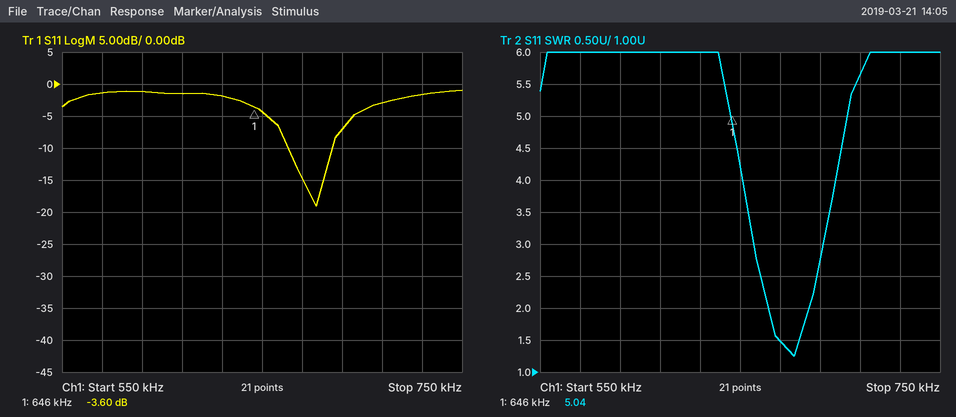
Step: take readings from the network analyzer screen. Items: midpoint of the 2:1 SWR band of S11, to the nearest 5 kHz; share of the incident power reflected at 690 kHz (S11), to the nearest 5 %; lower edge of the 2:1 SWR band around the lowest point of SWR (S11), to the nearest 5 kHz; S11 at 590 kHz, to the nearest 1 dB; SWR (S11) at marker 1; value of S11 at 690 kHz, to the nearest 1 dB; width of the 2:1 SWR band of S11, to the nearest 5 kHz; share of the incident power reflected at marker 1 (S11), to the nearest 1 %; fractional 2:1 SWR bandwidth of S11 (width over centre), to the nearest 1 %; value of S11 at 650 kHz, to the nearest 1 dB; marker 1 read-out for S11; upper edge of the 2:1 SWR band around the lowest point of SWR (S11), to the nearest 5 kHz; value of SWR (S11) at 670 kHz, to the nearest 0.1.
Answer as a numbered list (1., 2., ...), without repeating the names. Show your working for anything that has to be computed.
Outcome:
1. 675 kHz
2. 10^(-7/10) ≈ 20 %
3. 665 kHz
4. -1 dB
5. 5.04
6. -7 dB
7. 685 kHz − 665 kHz = 20 kHz
8. 10^(-3.6/10) ≈ 44 %
9. 20 kHz / 675 kHz ≈ 3 %
10. -4 dB
11. -3.60 dB
12. 685 kHz
13. 1.5
